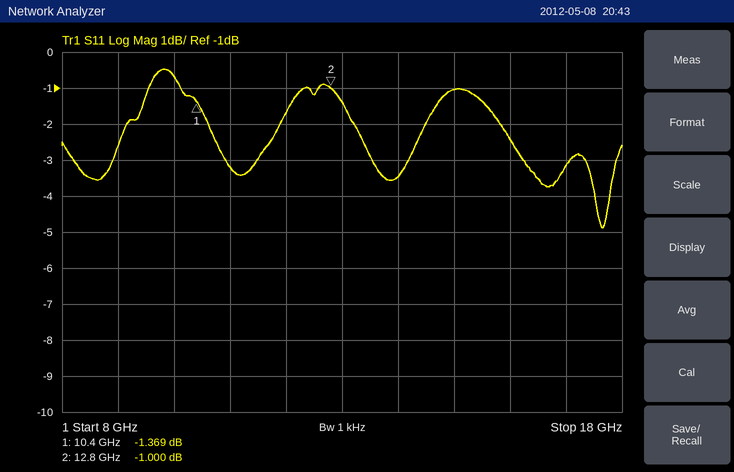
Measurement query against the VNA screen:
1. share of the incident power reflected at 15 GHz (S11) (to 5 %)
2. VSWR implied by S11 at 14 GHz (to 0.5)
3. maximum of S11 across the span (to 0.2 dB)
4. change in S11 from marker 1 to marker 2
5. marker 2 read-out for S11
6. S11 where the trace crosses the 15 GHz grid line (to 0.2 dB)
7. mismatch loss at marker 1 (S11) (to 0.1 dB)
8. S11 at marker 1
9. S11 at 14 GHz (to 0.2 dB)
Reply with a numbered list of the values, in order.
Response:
1. 80 %
2. 5.0
3. -0.4 dB
4. 0.369 dB
5. -1.000 dB
6. -1.0 dB
7. 5.7 dB
8. -1.369 dB
9. -3.4 dB
